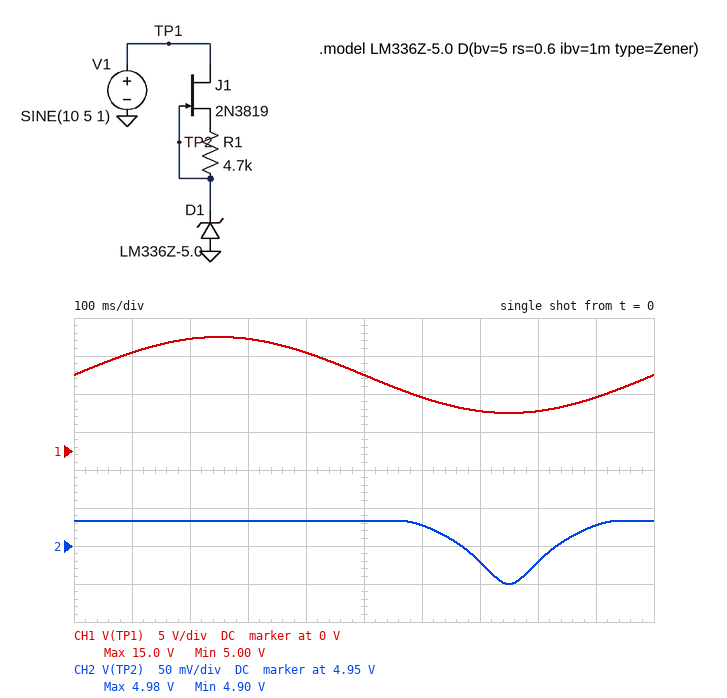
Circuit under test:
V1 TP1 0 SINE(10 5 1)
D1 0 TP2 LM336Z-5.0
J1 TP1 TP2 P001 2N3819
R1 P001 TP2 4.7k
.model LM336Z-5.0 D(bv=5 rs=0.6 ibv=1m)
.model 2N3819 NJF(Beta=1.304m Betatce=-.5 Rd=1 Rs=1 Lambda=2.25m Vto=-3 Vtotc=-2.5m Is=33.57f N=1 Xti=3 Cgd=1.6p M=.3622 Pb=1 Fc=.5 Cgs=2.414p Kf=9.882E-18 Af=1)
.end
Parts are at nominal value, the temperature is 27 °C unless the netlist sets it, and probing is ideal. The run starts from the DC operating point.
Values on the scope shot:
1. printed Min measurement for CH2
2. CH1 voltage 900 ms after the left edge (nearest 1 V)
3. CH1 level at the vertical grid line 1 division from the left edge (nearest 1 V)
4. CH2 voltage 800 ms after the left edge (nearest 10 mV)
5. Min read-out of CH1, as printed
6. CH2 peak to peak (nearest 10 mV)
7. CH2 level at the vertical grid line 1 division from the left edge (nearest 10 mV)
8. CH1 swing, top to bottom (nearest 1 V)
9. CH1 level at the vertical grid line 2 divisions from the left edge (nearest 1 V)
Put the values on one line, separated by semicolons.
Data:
4.90 V; 7 V; 13 V; 4.93 V; 5.00 V; 80 mV; 4.98 V; 10 V; 15 V
